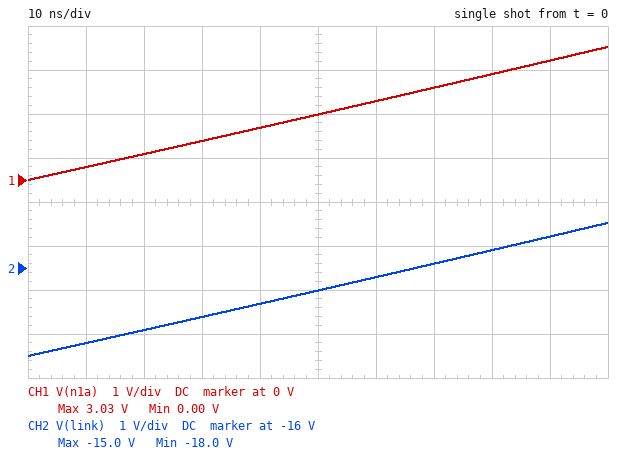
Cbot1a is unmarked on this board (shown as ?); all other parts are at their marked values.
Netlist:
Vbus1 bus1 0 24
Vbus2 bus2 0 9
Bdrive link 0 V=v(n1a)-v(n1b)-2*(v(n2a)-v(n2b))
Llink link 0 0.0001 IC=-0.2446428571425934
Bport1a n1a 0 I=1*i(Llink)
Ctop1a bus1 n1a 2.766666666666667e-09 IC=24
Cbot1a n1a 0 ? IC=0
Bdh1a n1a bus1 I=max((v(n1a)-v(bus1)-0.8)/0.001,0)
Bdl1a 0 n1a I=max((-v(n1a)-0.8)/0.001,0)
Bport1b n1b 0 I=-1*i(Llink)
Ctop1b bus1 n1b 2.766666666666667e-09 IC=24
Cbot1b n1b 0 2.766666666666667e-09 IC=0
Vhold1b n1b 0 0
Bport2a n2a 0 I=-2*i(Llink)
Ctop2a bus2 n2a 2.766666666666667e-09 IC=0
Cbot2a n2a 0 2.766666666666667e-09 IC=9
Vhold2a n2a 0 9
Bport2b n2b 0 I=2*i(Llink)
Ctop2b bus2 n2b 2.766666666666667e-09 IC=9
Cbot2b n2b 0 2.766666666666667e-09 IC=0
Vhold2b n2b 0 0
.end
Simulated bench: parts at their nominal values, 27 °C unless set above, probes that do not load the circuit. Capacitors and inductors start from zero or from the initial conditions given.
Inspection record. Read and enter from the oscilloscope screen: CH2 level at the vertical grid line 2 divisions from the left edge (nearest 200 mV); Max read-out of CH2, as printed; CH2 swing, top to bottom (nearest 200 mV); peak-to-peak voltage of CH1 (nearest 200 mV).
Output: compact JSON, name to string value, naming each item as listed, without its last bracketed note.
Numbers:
{"CH2 level at the vertical grid line 2 divisions from the left edge": "-17.4 V", "Max read-out of CH2, as printed": "-15.0 V", "CH2 swing, top to bottom": "3.0 V", "peak-to-peak voltage of CH1": "3.0 V"}
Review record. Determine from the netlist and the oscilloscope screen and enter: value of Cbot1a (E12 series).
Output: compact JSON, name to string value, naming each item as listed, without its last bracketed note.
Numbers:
{"value of Cbot1a": "5.6 nF"}
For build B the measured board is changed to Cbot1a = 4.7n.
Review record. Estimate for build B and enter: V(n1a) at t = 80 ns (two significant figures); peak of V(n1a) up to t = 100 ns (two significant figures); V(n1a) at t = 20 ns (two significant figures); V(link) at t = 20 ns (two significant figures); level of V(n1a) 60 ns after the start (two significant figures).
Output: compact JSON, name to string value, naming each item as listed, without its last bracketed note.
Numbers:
{"V(n1a) at t = 80 ns": "2.7 V", "peak of V(n1a) up to t = 100 ns": "3.4 V", "V(n1a) at t = 20 ns": "660 mV", "V(link) at t = 20 ns": "-17 V", "level of V(n1a) 60 ns after the start": "2.0 V"}
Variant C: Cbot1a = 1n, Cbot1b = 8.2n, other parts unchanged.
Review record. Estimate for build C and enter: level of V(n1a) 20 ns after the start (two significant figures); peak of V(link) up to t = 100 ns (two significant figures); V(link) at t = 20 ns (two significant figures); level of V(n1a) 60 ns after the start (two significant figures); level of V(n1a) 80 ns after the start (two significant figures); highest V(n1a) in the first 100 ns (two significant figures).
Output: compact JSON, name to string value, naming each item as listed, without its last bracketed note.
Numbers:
{"level of V(n1a) 20 ns after the start": "1.3 V", "peak of V(link) up to t = 100 ns": "-11 V", "V(link) at t = 20 ns": "-17 V", "level of V(n1a) 60 ns after the start": "4.0 V", "level of V(n1a) 80 ns after the start": "5.3 V", "highest V(n1a) in the first 100 ns": "6.7 V"}
